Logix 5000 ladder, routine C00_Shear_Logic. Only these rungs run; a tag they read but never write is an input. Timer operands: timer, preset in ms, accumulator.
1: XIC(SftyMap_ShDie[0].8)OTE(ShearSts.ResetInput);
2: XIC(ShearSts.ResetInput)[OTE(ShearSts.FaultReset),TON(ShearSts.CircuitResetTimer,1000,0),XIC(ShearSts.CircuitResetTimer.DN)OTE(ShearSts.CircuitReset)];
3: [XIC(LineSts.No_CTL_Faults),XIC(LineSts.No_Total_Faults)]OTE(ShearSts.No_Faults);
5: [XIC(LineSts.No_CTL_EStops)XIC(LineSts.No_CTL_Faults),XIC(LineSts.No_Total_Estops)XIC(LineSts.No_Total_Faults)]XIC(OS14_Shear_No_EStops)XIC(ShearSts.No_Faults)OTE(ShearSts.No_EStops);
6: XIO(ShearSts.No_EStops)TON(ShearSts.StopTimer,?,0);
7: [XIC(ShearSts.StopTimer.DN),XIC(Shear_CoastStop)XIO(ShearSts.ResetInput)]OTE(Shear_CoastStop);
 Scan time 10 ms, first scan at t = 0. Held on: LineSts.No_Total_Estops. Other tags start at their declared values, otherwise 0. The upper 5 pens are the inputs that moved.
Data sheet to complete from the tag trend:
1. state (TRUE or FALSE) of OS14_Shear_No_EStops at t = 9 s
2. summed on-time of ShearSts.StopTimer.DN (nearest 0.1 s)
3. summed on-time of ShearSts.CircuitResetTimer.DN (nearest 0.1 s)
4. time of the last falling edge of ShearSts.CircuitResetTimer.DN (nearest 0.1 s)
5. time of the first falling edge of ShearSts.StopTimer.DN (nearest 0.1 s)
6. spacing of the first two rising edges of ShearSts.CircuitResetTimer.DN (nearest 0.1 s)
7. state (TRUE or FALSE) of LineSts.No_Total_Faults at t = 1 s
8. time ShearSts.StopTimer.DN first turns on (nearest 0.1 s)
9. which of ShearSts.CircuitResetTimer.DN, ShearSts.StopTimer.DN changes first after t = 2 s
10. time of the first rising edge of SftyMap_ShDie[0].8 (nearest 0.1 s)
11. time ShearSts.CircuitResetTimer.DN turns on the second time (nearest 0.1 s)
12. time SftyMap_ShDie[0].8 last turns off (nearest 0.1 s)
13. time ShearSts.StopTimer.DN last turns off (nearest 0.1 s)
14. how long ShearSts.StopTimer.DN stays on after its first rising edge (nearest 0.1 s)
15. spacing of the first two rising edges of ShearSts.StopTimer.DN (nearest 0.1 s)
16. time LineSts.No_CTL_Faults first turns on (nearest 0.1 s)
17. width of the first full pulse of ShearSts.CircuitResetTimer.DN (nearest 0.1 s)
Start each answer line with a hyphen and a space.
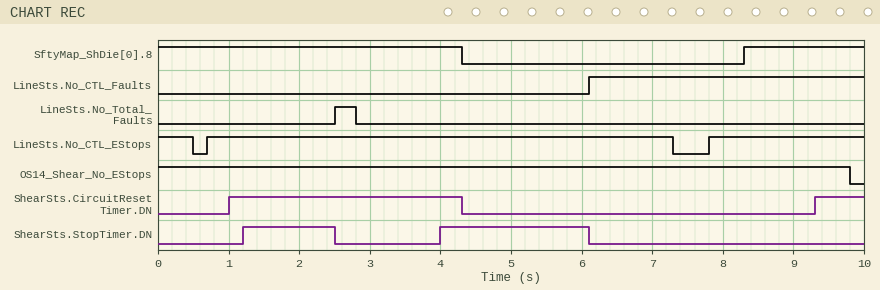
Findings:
- TRUE
- 3.4 s
- 4.0 s
- 4.3 s
- 2.5 s
- 8.3 s
- FALSE
- 1.2 s
- ShearSts.StopTimer.DN
- 8.3 s
- 9.3 s
- 4.3 s
- 6.1 s
- 1.3 s
- 2.8 s
- 6.1 s
- 3.3 s
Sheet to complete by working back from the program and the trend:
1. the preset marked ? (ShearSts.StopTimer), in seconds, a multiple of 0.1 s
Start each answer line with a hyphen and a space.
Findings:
- 1.2 s
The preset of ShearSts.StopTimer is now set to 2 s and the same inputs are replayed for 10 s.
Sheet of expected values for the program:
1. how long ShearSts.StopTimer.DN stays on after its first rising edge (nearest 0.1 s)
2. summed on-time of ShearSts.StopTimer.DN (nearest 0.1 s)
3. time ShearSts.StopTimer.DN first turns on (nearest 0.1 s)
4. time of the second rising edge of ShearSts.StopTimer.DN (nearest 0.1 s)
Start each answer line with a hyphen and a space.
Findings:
- 0.5 s
- 1.8 s
- 2.0 s
- 4.8 s
